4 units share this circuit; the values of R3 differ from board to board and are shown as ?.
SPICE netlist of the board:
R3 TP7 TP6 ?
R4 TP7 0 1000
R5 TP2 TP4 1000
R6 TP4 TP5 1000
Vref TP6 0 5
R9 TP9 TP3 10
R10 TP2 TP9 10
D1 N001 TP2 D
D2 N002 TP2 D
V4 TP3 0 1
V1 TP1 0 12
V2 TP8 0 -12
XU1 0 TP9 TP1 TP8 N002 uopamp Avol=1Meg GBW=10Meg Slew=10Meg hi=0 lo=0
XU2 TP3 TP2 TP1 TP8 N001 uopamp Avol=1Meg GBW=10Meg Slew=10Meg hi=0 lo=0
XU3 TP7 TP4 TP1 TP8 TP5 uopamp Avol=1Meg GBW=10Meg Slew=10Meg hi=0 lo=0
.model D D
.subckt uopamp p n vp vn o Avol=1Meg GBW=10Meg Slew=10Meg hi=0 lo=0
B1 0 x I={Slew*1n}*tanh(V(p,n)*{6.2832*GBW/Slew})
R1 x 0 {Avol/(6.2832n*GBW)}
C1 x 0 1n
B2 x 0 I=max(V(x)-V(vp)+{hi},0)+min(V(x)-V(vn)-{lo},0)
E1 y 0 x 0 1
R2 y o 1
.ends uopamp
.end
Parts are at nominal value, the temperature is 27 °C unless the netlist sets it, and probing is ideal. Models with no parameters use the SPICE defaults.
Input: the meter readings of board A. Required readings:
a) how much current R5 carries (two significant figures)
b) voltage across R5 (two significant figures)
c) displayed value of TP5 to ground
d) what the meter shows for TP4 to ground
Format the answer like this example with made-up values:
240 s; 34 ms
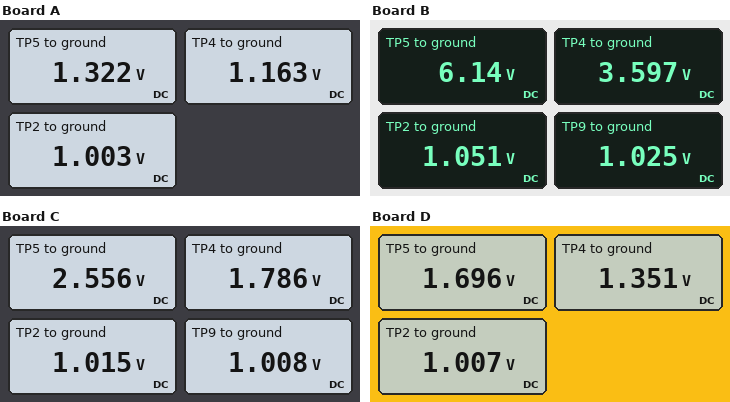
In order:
160 µA; 160 mV; 1.322 V; 1.163 V
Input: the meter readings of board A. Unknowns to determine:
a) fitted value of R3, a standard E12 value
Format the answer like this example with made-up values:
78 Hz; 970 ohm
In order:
3.3 kΩ
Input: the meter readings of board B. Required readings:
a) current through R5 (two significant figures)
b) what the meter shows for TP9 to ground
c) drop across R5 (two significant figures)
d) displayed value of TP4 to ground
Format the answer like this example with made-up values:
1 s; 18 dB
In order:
2.5 mA; 1.025 V; 2.5 V; 3.597 V
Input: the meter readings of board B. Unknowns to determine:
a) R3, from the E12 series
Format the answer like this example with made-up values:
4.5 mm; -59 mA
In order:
390 Ω
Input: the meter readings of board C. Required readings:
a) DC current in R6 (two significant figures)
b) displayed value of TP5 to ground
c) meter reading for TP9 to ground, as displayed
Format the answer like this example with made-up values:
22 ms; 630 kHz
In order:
770 µA; 2.556 V; 1.008 V
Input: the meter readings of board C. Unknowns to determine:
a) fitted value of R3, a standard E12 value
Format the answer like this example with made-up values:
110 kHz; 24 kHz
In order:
1.8 kΩ
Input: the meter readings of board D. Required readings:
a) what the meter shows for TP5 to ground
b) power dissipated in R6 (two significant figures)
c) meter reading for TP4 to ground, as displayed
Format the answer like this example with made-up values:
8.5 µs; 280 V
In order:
1.696 V; 120 µW; 1.351 V
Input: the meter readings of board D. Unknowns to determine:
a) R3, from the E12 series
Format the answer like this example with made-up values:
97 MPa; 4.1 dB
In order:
2.7 kΩ
